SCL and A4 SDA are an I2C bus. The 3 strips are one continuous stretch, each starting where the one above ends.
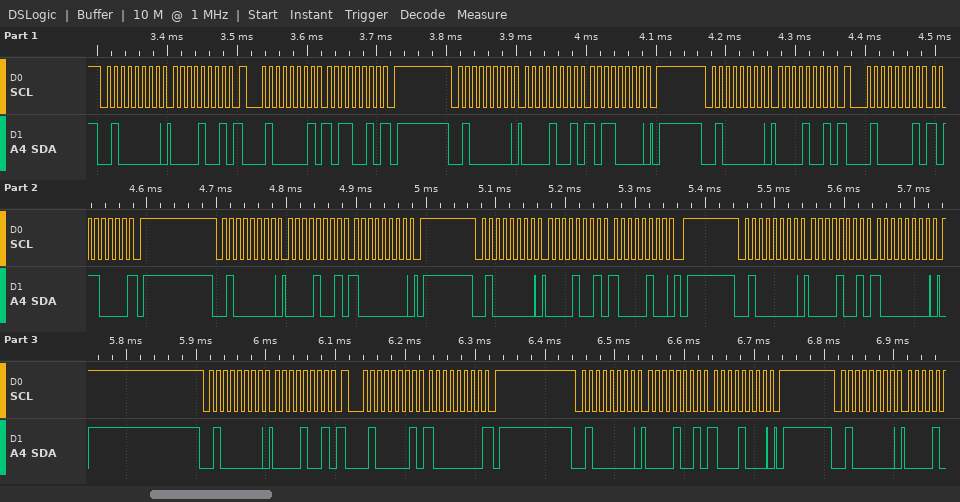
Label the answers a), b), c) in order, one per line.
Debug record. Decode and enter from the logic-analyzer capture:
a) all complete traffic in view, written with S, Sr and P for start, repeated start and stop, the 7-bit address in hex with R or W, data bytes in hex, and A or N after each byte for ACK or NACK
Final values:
a) S 20W A 09 A Sr 20R A B2 N P S 20W A 09 A B0 A P S 20W A 09 A Sr 20R A B0 N P S 20W A 09 A 80 A P S 20W A 09 A 84 A P S 20W A 09 A 80 A P S 20W A 09 A Sr 20R A 80 N P S 20W A 09 A 88 A P S 20W A
